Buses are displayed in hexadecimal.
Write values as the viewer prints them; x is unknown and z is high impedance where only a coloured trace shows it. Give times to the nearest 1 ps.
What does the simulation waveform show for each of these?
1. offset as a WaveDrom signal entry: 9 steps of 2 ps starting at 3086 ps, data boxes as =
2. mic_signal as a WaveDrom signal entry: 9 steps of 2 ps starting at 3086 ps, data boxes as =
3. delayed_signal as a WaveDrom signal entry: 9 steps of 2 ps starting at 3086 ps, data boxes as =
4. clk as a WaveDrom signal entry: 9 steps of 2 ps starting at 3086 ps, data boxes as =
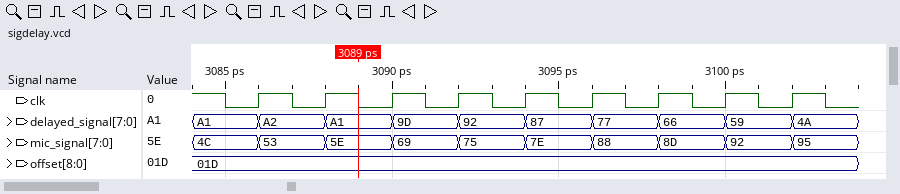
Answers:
{name: 'offset', wave: '=........', data: '01D'}
{name: 'mic_signal', wave: '=========', data: '53 5E 69 75 7E 88 8D 92 95'}
{name: 'delayed_signal', wave: '=========', data: 'A2 A1 9D 92 87 77 66 59 4A'}
{name: 'clk', wave: 'p........'}
